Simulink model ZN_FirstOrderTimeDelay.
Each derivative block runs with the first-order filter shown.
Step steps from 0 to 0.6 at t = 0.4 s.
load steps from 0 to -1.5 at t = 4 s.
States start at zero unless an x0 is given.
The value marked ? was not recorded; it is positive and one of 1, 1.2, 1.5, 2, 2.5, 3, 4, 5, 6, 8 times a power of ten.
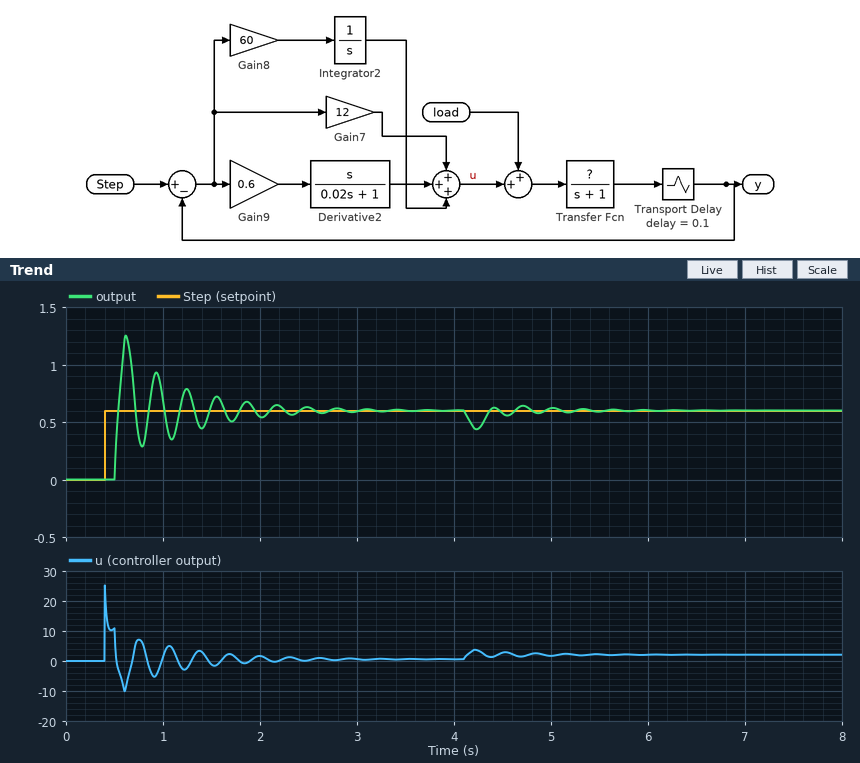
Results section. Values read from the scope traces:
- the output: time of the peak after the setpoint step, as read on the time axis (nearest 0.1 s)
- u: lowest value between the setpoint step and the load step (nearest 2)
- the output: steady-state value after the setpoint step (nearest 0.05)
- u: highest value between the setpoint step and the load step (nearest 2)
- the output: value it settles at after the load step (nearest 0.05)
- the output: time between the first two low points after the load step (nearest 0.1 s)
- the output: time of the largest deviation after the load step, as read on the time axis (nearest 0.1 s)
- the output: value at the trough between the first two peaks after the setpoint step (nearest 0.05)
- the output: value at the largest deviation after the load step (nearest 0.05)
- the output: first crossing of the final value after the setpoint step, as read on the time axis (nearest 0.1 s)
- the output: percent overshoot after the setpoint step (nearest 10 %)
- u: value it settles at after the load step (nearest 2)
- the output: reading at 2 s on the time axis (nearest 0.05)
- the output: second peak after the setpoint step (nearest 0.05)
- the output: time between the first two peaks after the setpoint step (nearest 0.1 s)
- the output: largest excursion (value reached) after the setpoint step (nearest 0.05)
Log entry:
0.6 s
-10
0.60
26
0.60
0.3 s
4.2 s
0.30
0.45
0.5 s
110 %
2
0.55
0.95
0.3 s
1.25
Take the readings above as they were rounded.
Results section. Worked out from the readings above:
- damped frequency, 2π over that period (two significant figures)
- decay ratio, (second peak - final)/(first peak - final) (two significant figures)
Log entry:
21 rad/s
0.54
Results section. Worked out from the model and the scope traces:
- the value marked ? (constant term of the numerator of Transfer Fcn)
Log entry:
1
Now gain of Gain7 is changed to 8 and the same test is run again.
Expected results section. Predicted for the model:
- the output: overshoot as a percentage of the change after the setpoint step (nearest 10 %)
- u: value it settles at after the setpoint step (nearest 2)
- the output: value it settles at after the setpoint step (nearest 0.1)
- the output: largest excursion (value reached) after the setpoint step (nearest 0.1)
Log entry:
70 %
0
0.6
1.0
